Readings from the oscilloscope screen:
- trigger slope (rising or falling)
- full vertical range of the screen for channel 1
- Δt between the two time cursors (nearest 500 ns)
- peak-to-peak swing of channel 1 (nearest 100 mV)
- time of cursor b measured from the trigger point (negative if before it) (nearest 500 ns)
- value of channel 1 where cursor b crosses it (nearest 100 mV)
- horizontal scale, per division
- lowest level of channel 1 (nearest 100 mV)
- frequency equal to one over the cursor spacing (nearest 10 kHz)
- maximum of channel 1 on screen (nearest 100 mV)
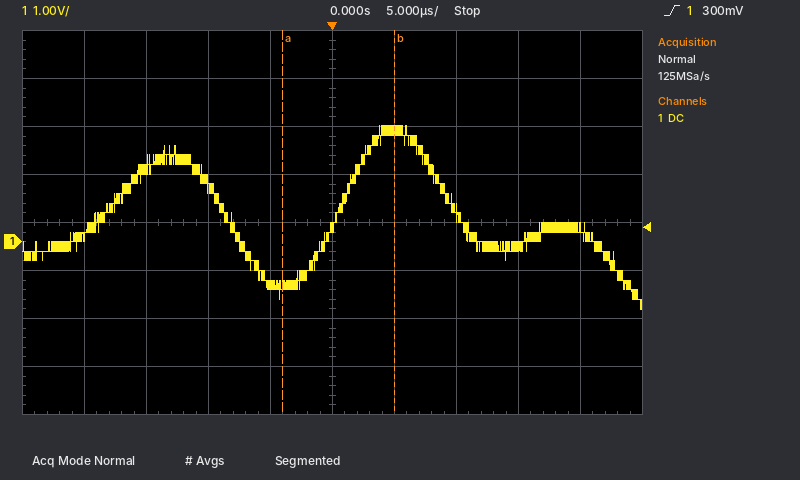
rising
8 V
9.0 µs
3.8 V
+5.0 µs
2.3 V
5 µs
-1.4 V
110 kHz
2.4 V
